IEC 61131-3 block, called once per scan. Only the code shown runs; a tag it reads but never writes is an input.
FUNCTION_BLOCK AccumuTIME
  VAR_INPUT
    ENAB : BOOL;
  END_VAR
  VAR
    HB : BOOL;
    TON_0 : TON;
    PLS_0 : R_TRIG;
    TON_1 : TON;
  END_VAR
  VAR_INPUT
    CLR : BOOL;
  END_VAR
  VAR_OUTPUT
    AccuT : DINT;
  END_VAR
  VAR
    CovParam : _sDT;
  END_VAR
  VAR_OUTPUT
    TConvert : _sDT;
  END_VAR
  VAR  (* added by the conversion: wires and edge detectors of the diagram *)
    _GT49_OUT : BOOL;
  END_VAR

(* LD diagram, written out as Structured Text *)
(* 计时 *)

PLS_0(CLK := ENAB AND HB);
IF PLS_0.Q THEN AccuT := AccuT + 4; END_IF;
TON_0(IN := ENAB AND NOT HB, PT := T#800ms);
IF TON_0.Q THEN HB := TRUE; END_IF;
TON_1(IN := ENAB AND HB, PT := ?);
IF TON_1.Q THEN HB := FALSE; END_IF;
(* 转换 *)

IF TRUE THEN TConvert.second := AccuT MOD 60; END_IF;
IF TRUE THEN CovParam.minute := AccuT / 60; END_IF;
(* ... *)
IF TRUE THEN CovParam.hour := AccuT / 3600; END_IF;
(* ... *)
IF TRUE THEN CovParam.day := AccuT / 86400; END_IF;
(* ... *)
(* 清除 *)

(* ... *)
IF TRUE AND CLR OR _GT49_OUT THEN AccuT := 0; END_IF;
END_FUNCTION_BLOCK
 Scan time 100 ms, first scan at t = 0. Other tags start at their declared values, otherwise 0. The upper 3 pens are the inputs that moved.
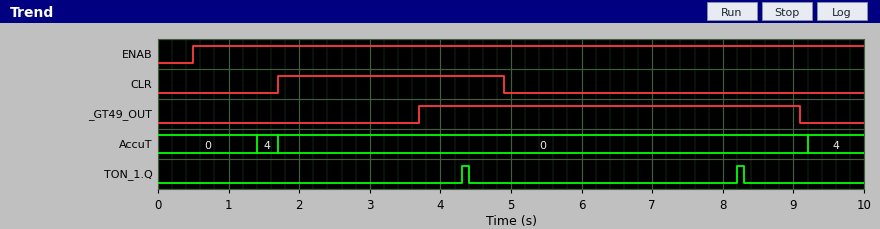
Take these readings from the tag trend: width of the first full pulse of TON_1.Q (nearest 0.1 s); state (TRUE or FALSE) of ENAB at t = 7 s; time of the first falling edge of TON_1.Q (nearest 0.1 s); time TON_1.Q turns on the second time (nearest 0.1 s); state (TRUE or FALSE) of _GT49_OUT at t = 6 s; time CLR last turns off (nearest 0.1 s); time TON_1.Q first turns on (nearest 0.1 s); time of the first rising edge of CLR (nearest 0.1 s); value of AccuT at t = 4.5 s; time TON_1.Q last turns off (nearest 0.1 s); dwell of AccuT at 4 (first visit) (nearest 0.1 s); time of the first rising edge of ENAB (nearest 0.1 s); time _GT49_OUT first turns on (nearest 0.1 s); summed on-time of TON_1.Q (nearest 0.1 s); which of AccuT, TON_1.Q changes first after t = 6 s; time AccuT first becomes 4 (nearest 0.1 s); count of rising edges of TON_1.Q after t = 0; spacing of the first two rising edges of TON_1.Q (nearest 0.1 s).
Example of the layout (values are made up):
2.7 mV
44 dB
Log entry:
0.1 s
TRUE
4.4 s
8.2 s
TRUE
4.9 s
4.3 s
1.7 s
0
8.3 s
0.3 s
0.5 s
3.7 s
0.2 s
TON_1.Q
1.4 s
2
3.9 s
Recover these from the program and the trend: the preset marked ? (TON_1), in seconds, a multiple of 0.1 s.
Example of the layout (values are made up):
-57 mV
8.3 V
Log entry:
3.0 s
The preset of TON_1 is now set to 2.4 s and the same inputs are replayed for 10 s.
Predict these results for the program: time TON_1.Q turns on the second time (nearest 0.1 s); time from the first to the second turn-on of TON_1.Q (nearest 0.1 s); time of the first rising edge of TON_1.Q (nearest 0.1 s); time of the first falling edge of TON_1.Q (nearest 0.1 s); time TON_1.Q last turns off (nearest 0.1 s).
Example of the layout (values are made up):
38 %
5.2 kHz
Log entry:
7.0 s
3.3 s
3.7 s
3.8 s
7.1 s
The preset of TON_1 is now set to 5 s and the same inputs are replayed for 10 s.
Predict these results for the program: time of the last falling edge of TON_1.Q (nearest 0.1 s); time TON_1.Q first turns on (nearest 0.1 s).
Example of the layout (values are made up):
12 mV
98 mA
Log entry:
6.4 s
6.3 s
